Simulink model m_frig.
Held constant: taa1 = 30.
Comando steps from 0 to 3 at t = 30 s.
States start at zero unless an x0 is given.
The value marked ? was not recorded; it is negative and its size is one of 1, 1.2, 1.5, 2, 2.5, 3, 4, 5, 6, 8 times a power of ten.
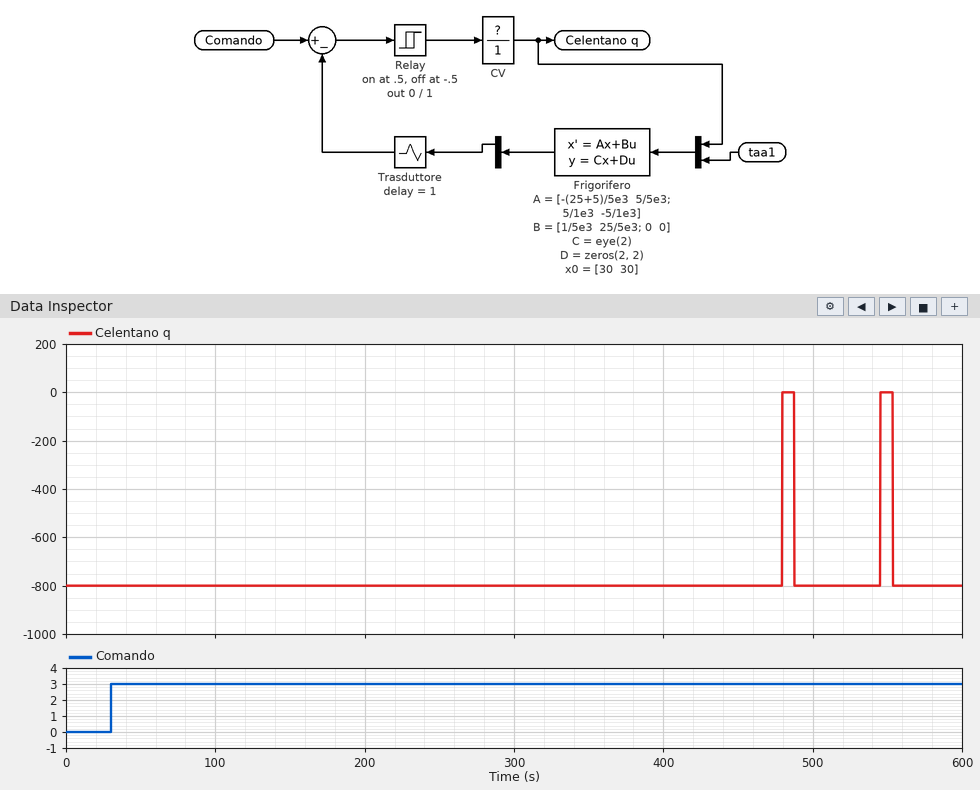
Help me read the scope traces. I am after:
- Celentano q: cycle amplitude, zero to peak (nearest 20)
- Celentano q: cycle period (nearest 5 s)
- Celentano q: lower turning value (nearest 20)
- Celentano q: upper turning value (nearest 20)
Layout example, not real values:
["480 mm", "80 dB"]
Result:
["400", "65 s", "-800", "0"]
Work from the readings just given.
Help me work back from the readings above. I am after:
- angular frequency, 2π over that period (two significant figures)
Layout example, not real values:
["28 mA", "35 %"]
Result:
["0.097 rad/s"]
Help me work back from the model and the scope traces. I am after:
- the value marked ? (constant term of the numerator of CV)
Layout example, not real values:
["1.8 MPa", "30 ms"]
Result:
["-800"]
